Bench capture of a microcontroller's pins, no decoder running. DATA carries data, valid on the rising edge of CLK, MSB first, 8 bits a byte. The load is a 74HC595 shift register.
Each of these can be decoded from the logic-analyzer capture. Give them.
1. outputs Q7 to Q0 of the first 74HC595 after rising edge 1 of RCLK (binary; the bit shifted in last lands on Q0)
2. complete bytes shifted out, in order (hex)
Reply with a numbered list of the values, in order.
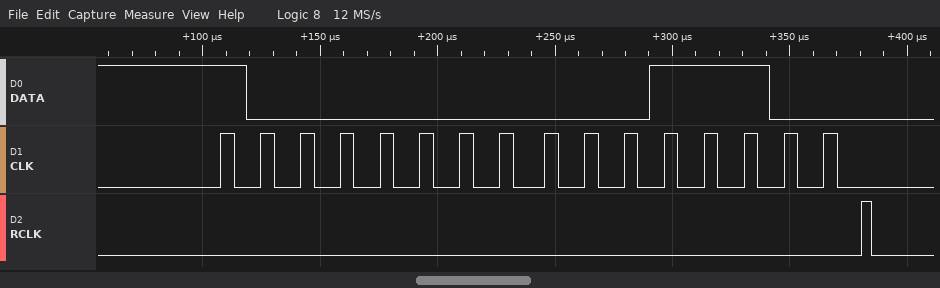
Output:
1. 00011100
2. 0x80 0x1C
